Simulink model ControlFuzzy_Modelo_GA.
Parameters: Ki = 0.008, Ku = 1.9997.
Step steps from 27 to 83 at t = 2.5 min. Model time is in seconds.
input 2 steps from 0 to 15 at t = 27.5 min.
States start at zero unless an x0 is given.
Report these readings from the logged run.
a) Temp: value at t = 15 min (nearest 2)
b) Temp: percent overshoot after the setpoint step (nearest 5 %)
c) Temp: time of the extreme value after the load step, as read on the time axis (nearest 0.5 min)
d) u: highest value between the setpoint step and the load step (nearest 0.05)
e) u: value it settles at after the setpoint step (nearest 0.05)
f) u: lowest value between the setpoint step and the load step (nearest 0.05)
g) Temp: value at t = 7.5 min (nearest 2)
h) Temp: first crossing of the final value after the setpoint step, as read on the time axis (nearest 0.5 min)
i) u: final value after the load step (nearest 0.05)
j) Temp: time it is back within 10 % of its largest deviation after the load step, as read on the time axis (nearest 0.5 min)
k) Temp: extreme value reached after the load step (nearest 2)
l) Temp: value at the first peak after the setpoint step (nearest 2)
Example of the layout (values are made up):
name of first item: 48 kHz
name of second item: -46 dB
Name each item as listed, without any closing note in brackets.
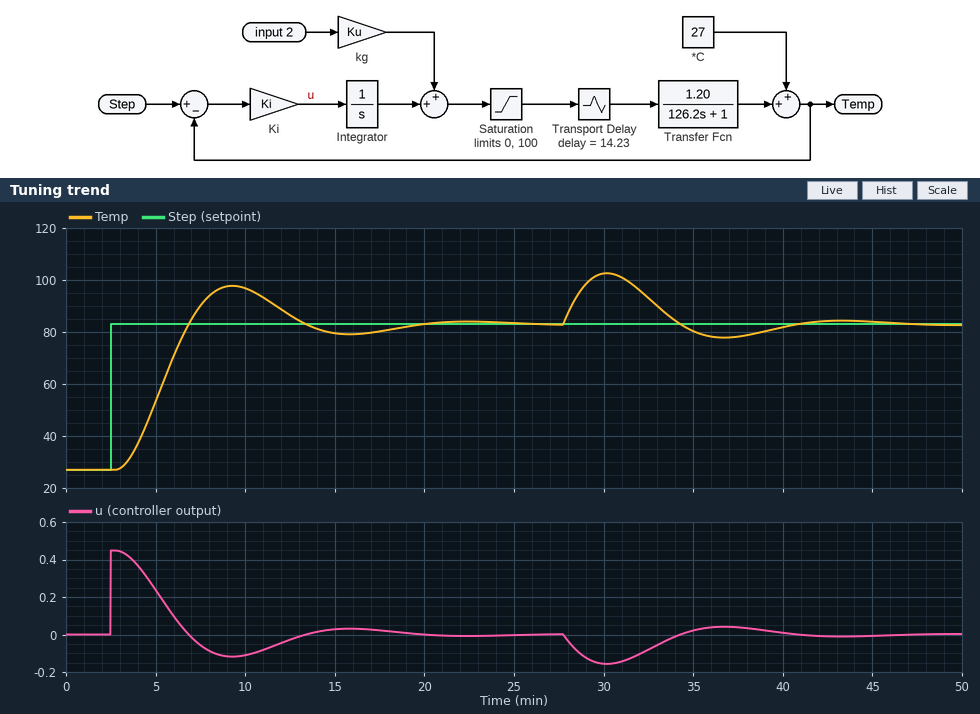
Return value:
Temp: value at t = 15 min: 80
Temp: percent overshoot after the setpoint step: 25 %
Temp: time of the extreme value after the load step, as read on the time axis: 30.0 min
u: highest value between the setpoint step and the load step: 0.45
u: value it settles at after the setpoint step: 0.00
u: lowest value between the setpoint step and the load step: -0.10
Temp: value at t = 7.5 min: 90
Temp: first crossing of the final value after the setpoint step, as read on the time axis: 7.0 min
u: final value after the load step: 0.00
Temp: time it is back within 10 % of its largest deviation after the load step, as read on the time axis: 39.5 min
Temp: extreme value reached after the load step: 102
Temp: value at the first peak after the setpoint step: 98
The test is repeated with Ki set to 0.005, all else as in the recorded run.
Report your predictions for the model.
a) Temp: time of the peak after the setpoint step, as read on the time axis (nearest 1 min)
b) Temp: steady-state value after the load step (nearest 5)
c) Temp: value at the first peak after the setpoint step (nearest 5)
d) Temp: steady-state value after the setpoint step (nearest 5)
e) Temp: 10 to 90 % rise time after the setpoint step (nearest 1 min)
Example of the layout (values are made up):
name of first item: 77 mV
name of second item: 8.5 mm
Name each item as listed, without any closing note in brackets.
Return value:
Temp: time of the peak after the setpoint step, as read on the time axis: 12 min
Temp: steady-state value after the load step: 85
Temp: value at the first peak after the setpoint step: 90
Temp: steady-state value after the setpoint step: 85
Temp: 10 to 90 % rise time after the setpoint step: 4 min
